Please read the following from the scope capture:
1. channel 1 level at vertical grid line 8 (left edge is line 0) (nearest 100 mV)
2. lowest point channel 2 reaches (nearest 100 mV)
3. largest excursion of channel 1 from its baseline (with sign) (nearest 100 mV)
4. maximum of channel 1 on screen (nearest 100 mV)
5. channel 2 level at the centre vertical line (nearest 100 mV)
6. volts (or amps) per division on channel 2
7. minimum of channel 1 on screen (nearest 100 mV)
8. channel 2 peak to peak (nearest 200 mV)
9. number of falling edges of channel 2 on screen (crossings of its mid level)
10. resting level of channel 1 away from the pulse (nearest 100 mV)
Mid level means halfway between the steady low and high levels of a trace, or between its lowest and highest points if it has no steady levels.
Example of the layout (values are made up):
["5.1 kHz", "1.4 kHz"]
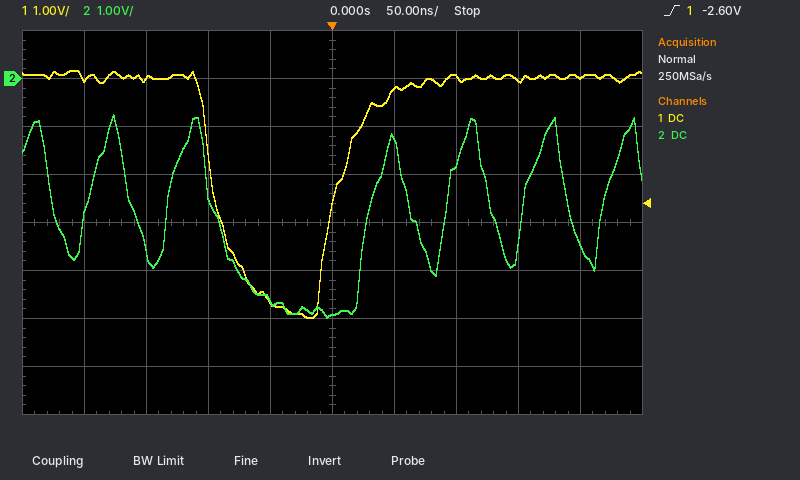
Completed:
["0.0 V", "-5.0 V", "-5.0 V", "200 mV", "-4.9 V", "1 V", "-5.0 V", "4.2 V", "6", "0.0 V"]
